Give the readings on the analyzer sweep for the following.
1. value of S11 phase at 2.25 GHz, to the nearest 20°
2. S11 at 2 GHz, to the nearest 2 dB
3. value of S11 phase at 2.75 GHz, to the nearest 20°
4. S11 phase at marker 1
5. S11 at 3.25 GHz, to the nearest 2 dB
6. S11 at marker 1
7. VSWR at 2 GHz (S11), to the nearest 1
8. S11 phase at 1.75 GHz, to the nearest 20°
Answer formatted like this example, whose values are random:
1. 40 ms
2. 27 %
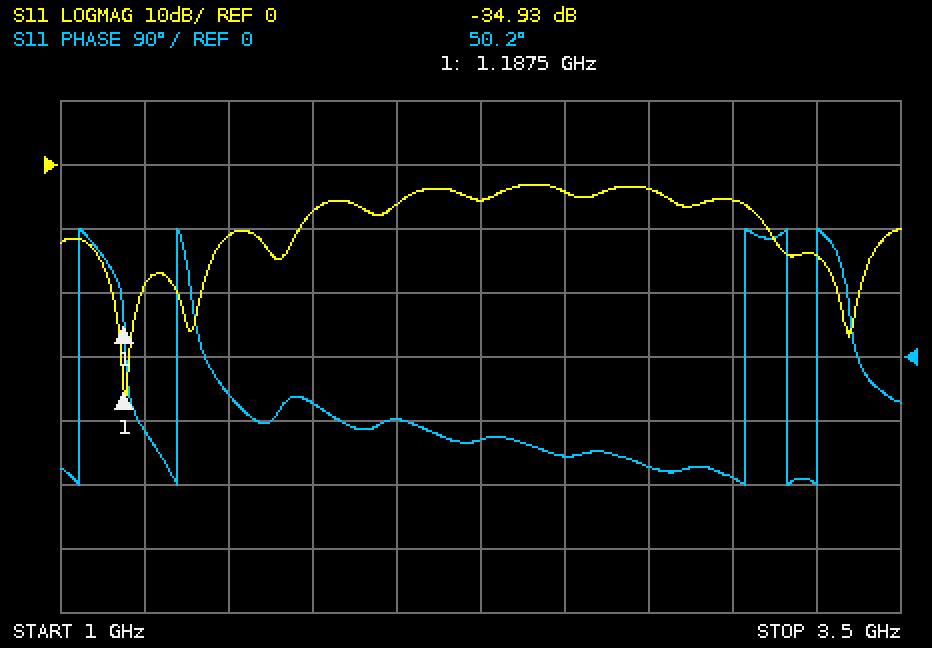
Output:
1. -120°
2. -6 dB
3. -160°
4. 50.2°
5. -14 dB
6. -34.93 dB
7. 3
8. -60°
